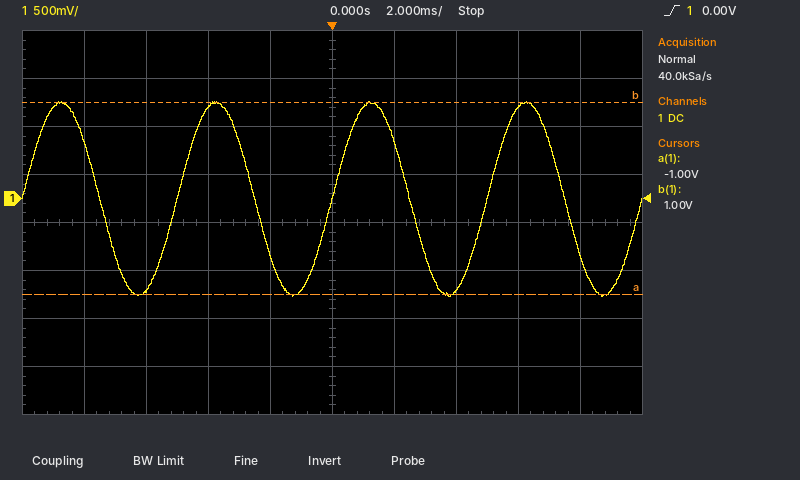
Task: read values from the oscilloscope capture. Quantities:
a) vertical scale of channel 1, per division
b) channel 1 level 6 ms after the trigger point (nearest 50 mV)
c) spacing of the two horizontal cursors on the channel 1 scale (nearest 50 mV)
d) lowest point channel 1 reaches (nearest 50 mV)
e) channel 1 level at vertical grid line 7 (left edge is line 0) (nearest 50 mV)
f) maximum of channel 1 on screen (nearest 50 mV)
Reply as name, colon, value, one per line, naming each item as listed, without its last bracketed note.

vertical scale of channel 1, per division: 500 mV
channel 1 level 6 ms after the trigger point: 950 mV
spacing of the two horizontal cursors on the channel 1 scale: 2.00 V
lowest point channel 1 reaches: -1.00 V
channel 1 level at vertical grid line 7 (left edge is line 0): -950 mV
maximum of channel 1 on screen: 1.00 V
